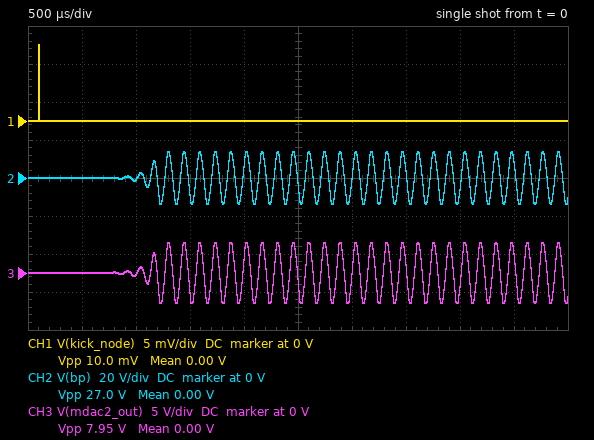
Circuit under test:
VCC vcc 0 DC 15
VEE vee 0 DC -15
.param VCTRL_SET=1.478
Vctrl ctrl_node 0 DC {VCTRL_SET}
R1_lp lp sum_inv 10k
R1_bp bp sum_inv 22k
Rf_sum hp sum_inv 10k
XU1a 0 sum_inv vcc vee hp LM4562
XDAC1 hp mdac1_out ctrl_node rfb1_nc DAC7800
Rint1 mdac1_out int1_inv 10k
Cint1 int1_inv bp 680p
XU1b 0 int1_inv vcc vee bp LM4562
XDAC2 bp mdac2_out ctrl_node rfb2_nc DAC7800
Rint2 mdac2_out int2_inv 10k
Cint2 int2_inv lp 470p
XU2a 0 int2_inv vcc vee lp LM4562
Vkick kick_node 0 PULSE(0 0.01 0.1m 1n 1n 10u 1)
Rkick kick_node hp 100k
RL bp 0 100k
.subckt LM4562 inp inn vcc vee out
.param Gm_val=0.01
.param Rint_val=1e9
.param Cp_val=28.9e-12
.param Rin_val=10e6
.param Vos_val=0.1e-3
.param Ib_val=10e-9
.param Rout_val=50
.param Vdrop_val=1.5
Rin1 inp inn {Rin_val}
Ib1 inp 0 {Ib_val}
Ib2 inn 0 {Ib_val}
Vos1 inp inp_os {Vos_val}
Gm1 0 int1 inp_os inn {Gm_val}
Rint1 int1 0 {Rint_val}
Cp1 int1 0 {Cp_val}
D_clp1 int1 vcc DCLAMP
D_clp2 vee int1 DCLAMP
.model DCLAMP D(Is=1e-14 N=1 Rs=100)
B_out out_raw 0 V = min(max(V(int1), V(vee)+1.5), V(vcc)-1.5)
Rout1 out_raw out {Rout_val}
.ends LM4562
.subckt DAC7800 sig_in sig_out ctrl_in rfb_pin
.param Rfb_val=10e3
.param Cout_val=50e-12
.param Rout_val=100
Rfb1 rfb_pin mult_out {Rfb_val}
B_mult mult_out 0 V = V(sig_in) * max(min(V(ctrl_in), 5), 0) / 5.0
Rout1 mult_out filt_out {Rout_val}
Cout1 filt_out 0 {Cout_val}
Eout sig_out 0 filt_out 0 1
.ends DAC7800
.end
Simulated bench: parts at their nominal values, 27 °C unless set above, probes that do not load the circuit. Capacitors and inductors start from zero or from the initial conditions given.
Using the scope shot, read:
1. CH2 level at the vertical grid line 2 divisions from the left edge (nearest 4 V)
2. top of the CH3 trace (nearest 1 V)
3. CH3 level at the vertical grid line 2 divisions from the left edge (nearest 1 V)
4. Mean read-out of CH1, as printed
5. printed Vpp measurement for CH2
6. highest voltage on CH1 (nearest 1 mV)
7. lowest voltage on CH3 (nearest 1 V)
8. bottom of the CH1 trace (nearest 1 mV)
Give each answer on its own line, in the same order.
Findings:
0 V
4 V
0 V
0.00 V
27.0 V
10 mV
-4 V
0 V
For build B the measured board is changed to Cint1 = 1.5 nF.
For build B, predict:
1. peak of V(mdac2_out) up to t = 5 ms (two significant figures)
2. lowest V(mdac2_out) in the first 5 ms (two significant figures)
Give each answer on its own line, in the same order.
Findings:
2.8 V
-2.8 V
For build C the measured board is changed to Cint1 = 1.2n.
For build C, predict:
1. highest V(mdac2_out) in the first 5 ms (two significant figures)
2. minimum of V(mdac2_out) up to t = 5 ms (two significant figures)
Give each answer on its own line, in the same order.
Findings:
3.2 V
-3.2 V
